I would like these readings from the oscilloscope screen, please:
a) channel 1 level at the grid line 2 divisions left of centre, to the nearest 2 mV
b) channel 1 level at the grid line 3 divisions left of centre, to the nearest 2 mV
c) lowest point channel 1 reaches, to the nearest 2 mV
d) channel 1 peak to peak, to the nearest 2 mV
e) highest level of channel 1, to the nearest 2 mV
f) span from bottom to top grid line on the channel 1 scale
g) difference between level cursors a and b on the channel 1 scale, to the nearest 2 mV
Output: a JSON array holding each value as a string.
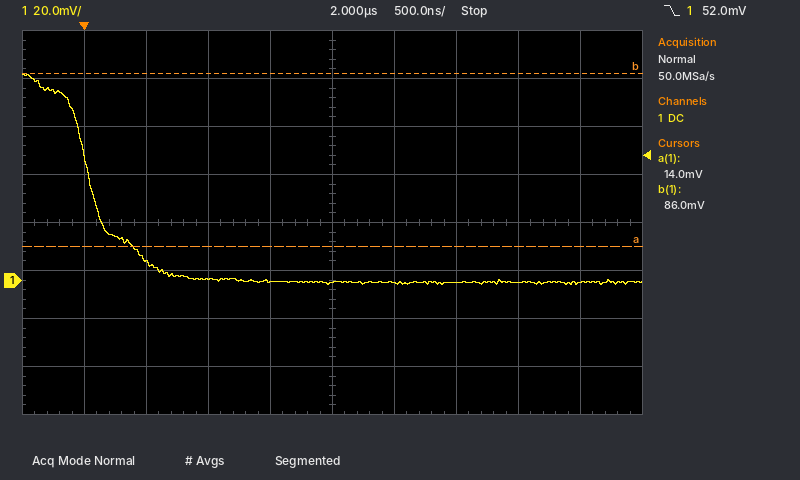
["0 mV", "8 mV", "-2 mV", "88 mV", "86 mV", "160 mV", "72 mV"]
